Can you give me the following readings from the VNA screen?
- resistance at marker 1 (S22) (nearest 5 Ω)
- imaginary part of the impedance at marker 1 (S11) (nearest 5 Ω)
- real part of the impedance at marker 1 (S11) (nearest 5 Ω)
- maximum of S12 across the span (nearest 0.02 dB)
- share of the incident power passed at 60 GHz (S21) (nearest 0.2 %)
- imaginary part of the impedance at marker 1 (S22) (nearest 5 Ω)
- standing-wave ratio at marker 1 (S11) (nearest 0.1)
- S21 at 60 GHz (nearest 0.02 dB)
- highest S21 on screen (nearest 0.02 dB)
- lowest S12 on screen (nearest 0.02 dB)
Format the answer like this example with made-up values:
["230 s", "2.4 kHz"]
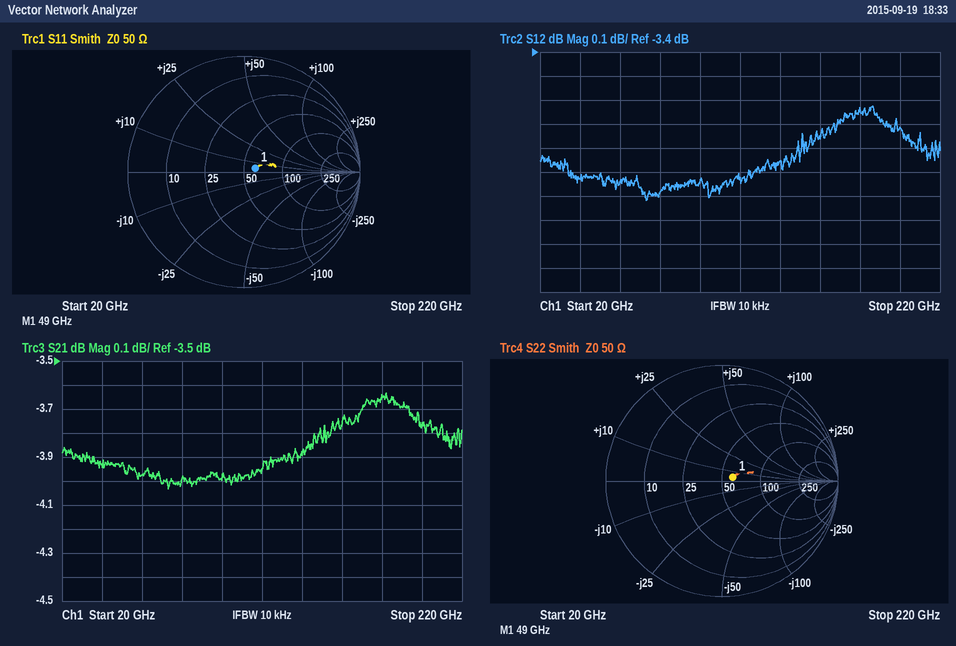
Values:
["60 Ω", "+5 Ω", "60 Ω", "-3.62 dB", "40.0 %", "+5 Ω", "1.2", "-3.98 dB", "-3.64 dB", "-4.02 dB"]
